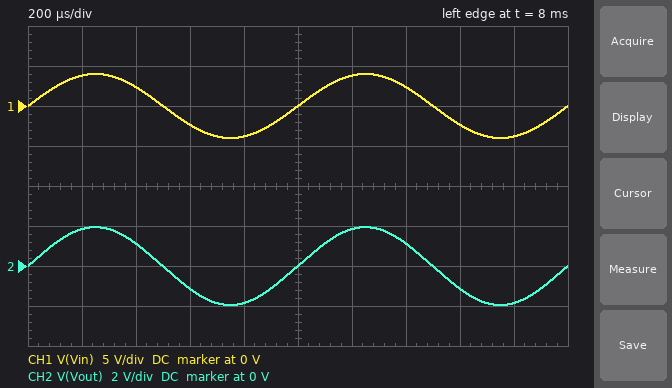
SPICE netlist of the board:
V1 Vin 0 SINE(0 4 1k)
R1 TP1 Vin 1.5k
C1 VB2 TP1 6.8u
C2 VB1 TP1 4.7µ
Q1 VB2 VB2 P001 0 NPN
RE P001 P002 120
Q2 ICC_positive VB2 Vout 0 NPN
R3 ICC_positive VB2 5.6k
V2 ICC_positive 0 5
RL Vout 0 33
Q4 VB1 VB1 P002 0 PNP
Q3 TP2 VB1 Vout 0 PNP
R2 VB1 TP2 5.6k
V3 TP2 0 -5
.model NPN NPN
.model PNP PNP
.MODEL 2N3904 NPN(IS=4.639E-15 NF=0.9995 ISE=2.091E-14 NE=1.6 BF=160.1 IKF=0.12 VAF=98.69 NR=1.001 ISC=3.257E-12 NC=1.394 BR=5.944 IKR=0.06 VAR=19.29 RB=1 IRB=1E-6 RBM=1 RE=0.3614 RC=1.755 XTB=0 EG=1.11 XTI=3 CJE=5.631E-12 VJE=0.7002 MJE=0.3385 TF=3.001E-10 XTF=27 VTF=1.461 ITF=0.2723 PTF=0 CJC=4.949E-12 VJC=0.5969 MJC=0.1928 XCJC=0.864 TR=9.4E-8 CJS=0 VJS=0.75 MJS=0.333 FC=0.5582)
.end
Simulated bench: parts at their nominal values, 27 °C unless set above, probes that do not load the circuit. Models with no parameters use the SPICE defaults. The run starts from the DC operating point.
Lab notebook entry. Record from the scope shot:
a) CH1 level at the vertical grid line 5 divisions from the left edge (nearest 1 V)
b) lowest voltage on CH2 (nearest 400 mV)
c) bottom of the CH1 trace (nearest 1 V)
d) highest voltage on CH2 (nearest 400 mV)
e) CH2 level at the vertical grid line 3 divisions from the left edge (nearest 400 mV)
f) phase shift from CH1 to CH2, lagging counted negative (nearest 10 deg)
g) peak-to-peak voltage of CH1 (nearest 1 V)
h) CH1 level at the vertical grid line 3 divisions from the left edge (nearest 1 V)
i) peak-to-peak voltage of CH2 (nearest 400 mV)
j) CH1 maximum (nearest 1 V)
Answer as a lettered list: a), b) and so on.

a) 0 V
b) -2.0 V
c) -4 V
d) 2.0 V
e) -1.2 V
f) 0 deg
g) 8 V
h) -2 V
i) 4.0 V
j) 4 V
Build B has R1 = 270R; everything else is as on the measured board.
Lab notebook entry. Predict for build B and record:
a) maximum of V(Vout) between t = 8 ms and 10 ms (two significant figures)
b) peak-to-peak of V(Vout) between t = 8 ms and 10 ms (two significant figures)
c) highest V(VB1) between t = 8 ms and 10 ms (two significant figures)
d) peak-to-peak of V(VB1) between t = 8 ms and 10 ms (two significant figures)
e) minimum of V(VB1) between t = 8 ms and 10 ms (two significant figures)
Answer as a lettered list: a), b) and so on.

a) 3.3 V
b) 6.6 V
c) 2.6 V
d) 6.8 V
e) -4.2 V
